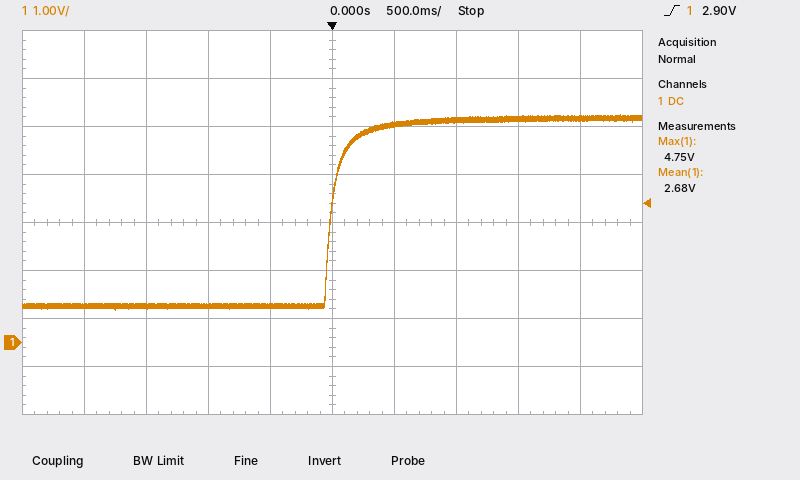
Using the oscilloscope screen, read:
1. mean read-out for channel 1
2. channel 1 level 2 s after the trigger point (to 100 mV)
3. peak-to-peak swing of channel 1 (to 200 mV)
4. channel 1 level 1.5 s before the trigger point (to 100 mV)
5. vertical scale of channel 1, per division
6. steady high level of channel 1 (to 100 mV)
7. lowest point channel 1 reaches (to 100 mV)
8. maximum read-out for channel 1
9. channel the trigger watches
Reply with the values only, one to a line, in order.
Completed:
2.68 V
4.7 V
4.0 V
800 mV
1 V
4.7 V
700 mV
4.75 V
channel 1
